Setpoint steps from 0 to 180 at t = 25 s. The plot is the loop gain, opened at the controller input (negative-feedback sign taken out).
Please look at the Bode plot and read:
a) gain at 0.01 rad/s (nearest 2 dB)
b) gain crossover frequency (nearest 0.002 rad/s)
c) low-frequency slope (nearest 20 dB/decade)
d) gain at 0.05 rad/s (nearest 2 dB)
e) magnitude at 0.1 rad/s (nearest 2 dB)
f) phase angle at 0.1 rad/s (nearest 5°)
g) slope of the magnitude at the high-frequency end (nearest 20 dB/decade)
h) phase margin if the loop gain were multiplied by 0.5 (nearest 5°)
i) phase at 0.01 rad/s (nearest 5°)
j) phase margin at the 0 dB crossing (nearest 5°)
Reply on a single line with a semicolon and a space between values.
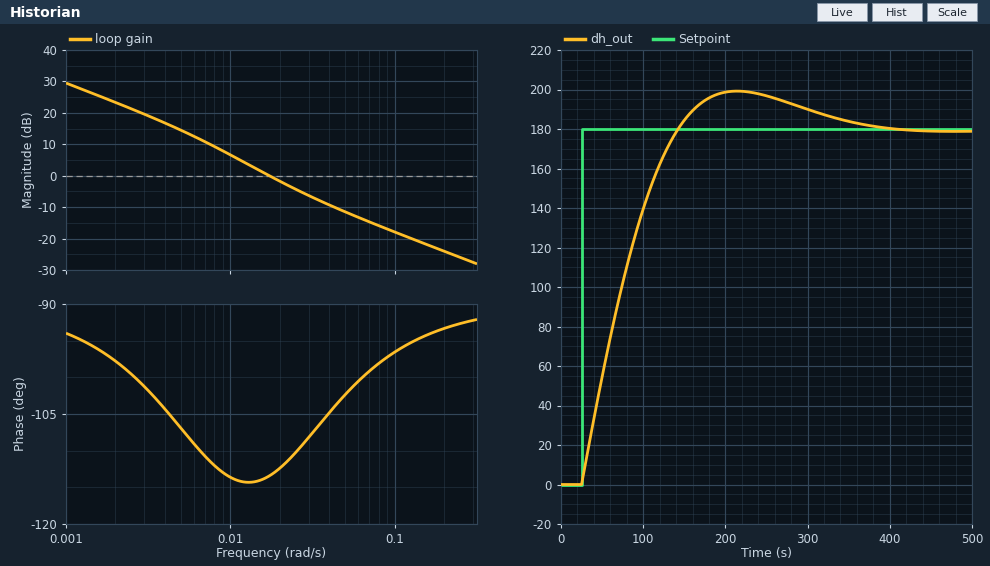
6 dB; 0.018 rad/s; -20 dB/decade; -12 dB; -18 dB; -95°; -20 dB/decade; 65°; -115°; 65°
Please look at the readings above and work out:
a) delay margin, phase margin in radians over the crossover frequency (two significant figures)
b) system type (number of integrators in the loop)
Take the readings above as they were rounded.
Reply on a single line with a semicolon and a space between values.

63 s; 1
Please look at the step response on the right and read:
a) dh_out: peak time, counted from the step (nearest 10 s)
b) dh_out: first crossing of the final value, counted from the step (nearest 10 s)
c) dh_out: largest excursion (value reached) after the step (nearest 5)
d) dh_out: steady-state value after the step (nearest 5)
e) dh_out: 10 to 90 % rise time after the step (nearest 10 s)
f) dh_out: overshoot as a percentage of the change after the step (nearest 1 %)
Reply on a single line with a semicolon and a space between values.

190 s; 120 s; 200; 180; 90 s; 11 %
